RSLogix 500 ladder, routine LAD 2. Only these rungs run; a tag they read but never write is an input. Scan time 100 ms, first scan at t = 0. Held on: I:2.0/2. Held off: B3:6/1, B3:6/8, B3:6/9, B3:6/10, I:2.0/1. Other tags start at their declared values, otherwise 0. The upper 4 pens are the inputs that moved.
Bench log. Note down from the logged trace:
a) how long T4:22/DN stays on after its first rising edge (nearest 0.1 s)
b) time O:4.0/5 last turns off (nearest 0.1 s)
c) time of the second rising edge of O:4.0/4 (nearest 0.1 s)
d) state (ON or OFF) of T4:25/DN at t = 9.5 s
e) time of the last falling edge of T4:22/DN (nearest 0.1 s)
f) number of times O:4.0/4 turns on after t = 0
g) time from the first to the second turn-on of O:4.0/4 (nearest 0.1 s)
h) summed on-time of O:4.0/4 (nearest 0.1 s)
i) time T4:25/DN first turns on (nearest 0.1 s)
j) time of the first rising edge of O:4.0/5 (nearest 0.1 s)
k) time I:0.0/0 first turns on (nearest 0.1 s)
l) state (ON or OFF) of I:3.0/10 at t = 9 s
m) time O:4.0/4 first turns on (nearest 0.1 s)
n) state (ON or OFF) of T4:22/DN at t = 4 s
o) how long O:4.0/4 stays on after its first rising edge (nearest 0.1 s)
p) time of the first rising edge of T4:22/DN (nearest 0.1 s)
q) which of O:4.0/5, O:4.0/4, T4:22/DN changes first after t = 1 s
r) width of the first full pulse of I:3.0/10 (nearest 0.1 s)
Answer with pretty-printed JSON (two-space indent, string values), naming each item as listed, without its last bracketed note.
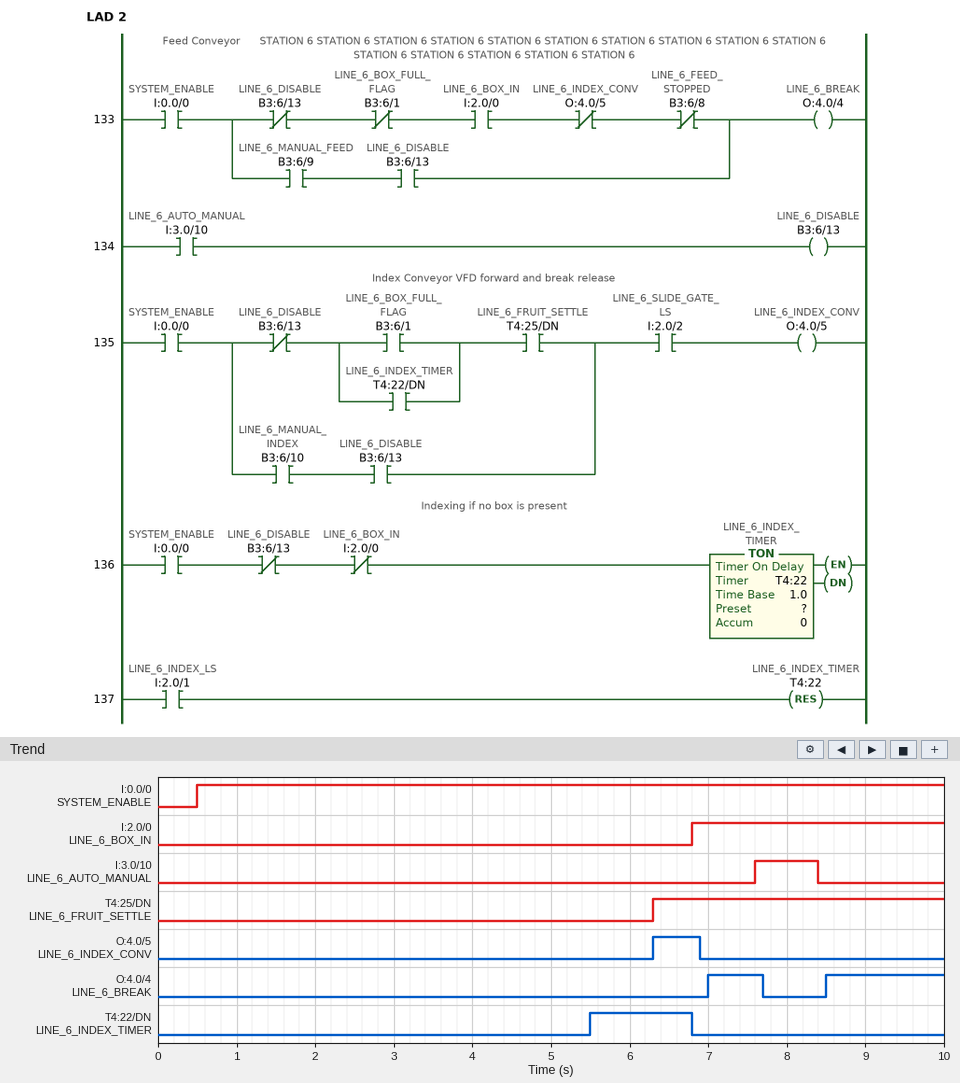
{
  "how long T4:22/DN stays on after its first rising edge": "1.3 s",
  "time O:4.0/5 last turns off": "6.9 s",
  "time of the second rising edge of O:4.0/4": "8.5 s",
  "state (ON or OFF) of T4:25/DN at t = 9.5 s": "ON",
  "time of the last falling edge of T4:22/DN": "6.8 s",
  "number of times O:4.0/4 turns on after t = 0": "2",
  "time from the first to the second turn-on of O:4.0/4": "1.5 s",
  "summed on-time of O:4.0/4": "2.2 s",
  "time T4:25/DN first turns on": "6.3 s",
  "time of the first rising edge of O:4.0/5": "6.3 s",
  "time I:0.0/0 first turns on": "0.5 s",
  "state (ON or OFF) of I:3.0/10 at t = 9 s": "OFF",
  "time O:4.0/4 first turns on": "7.0 s",
  "state (ON or OFF) of T4:22/DN at t = 4 s": "OFF",
  "how long O:4.0/4 stays on after its first rising edge": "0.7 s",
  "time of the first rising edge of T4:22/DN": "5.5 s",
  "which of O:4.0/5, O:4.0/4, T4:22/DN changes first after t = 1 s": "T4:22/DN",
  "width of the first full pulse of I:3.0/10": "0.8 s"
}
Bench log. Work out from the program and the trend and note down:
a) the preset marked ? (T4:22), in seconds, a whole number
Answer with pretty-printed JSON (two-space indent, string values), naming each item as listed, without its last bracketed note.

{
  "the preset marked ? (T4:22), in seconds, a whole number": "5 s"
}
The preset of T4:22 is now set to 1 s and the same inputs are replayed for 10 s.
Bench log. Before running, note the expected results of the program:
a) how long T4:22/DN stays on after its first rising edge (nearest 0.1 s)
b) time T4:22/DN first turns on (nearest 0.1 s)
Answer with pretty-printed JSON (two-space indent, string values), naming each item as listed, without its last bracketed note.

{
  "how long T4:22/DN stays on after its first rising edge": "5.3 s",
  "time T4:22/DN first turns on": "1.5 s"
}
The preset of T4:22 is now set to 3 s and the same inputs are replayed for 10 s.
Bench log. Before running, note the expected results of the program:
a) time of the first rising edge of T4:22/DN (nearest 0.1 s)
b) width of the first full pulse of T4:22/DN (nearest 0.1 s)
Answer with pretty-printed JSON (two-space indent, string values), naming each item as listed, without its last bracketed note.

{
  "time of the first rising edge of T4:22/DN": "3.5 s",
  "width of the first full pulse of T4:22/DN": "3.3 s"
}
